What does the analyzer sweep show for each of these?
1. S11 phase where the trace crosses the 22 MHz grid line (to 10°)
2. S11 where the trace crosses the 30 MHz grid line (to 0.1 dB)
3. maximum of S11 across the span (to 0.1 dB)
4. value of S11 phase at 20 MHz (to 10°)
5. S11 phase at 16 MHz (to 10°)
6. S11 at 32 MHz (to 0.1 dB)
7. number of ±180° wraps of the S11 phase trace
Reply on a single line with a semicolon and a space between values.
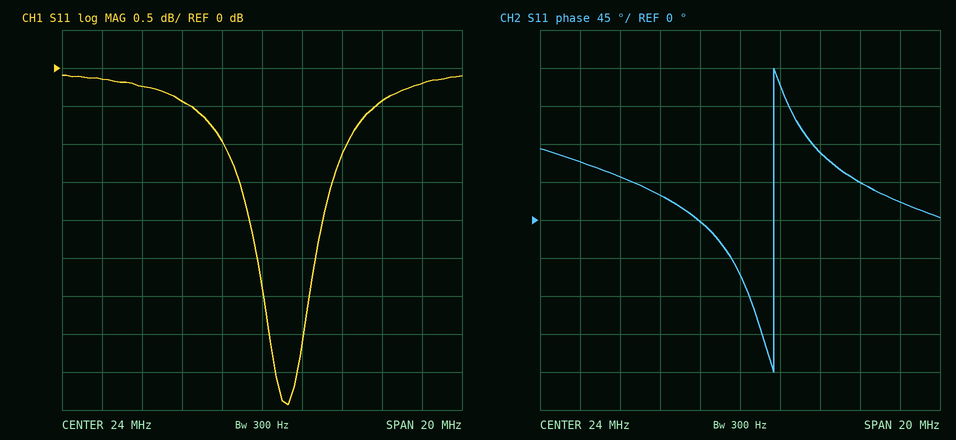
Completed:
0°; -0.4 dB; -0.1 dB; 30°; 70°; -0.2 dB; 1
